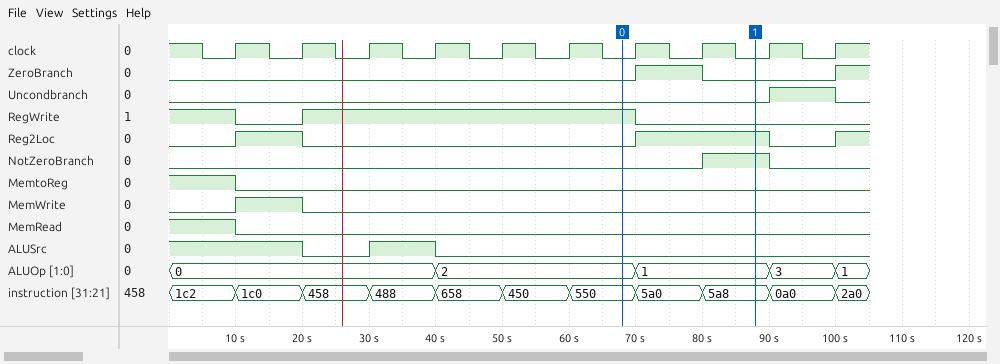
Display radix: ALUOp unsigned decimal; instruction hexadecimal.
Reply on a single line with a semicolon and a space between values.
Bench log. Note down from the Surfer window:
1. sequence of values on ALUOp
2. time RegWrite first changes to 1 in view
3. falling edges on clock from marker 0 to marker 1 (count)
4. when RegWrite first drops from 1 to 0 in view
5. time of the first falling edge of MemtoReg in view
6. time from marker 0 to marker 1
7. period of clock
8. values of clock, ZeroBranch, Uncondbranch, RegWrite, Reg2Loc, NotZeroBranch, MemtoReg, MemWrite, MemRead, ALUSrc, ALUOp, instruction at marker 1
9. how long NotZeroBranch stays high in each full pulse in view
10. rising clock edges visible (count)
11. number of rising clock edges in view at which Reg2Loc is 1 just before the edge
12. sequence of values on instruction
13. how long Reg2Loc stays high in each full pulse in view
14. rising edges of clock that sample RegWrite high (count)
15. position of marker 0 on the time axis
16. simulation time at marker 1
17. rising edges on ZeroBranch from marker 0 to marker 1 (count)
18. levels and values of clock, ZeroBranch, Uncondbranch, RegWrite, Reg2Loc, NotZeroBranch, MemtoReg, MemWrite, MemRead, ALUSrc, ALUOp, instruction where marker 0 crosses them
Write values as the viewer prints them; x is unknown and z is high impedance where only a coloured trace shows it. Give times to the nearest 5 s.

0, 2, 1, 3, 1; 20 s; 2; 10 s; 10 s; 20 s; 10 s; clock=0, ZeroBranch=0, Uncondbranch=0, RegWrite=0, Reg2Loc=1, NotZeroBranch=1, MemtoReg=0, MemWrite=0, MemRead=0, ALUSrc=0, ALUOp=1, instruction=5a8; 10 s; 10; 3; 1c2, 1c0, 458, 488, 658, 450, 550, 5a0, 5a8, 0a0, 2a0; 10 s, 20 s; 6; 70 s; 90 s; 1; clock=0, ZeroBranch=0, Uncondbranch=0, RegWrite=1, Reg2Loc=0, NotZeroBranch=0, MemtoReg=0, MemWrite=0, MemRead=0, ALUSrc=0, ALUOp=2, instruction=550
